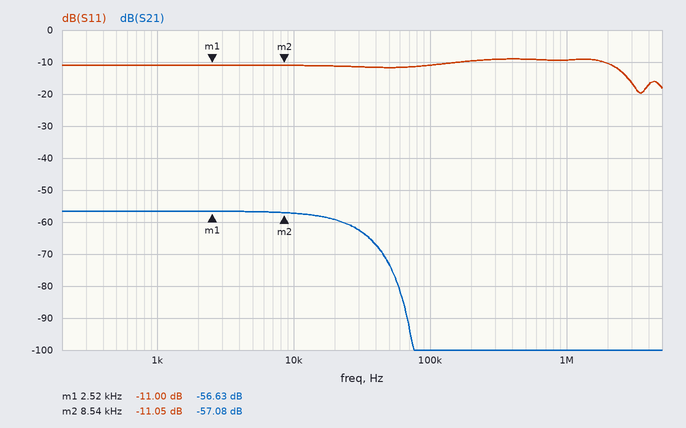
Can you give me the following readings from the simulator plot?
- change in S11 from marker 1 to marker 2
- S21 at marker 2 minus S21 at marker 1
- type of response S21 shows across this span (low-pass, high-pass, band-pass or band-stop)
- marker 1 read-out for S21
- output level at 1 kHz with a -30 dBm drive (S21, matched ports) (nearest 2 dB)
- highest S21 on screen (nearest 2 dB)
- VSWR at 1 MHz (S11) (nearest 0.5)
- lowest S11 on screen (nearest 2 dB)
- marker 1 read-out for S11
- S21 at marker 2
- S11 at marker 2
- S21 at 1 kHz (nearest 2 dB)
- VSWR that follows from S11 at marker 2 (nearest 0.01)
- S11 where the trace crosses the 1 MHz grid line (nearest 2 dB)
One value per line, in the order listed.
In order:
-0.05 dB
-0.45 dB
low-pass
-56.63 dB
-86 dBm
-56 dB
2.0
-20 dB
-11.00 dB
-57.08 dB
-11.05 dB
-56 dB
1.78
-10 dB
